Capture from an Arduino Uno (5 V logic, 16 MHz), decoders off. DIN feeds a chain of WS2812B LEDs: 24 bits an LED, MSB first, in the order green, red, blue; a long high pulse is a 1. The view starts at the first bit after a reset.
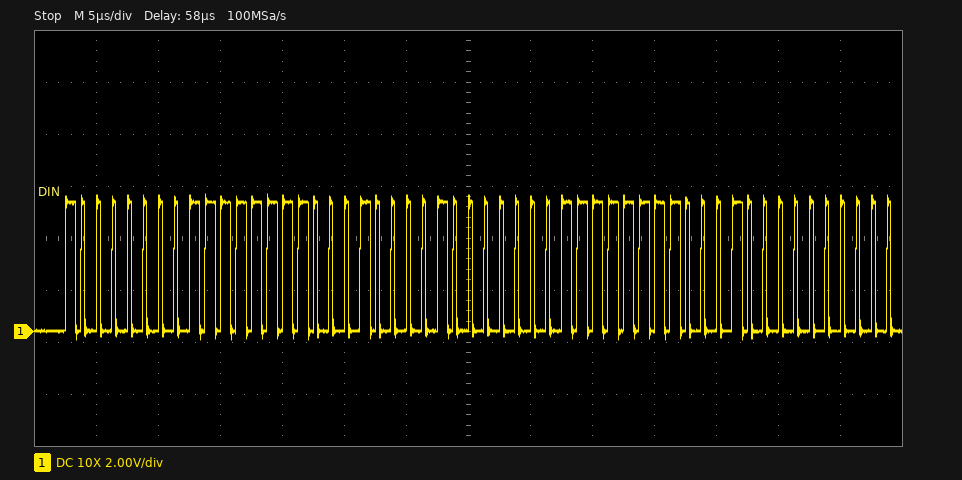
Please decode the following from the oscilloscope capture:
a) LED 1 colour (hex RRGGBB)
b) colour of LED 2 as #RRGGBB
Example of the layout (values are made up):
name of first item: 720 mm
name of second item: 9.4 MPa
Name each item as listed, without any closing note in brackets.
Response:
LED 1 colour: #FF8010
colour of LED 2 as #RRGGBB: #FF8010
